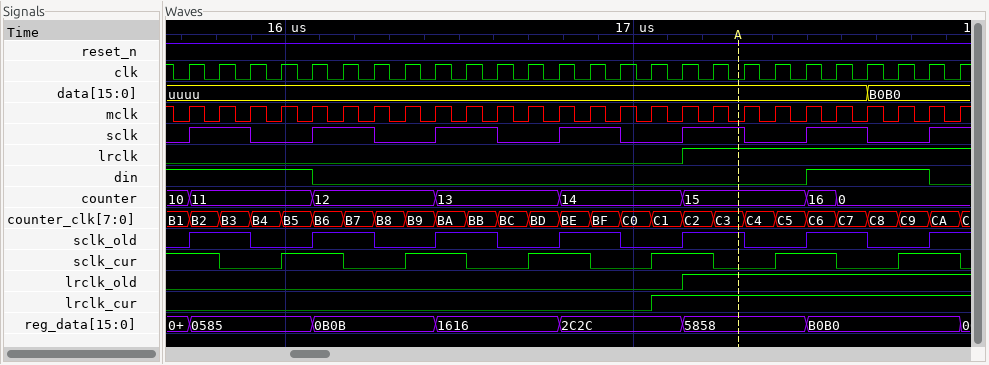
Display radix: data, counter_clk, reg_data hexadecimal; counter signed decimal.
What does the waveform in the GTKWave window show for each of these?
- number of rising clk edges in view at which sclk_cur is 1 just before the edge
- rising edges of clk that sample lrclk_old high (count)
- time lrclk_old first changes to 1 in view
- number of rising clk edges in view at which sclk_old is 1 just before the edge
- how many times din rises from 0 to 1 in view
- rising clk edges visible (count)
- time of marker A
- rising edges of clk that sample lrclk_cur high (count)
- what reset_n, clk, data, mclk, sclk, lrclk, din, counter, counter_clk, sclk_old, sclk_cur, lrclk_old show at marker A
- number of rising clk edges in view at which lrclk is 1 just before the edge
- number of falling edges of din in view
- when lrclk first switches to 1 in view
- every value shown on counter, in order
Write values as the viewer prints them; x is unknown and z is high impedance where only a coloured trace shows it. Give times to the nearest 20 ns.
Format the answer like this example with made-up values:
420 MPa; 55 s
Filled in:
14; 9; 17140 ns; 13; 1; 26; 17300 ns; 10; reset_n=1, clk=0, data=uuuu, mclk=0, sclk=1, lrclk=1, din=0, counter=15, counter_clk=C3, sclk_old=1, sclk_cur=0, lrclk_old=1; 9; 2; 17140 ns; 10, 11, 12, 13, 14, 15, 16, 0
